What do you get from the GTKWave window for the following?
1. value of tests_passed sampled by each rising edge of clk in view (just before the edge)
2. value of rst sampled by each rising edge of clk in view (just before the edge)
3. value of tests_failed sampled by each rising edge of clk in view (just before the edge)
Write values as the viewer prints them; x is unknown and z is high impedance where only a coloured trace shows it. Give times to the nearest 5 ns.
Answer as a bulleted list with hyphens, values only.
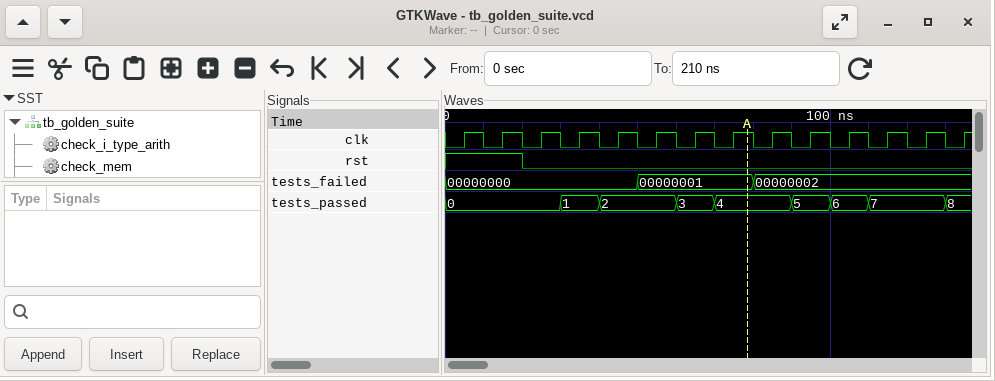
- 0, 0, 0, 1, 2, 2, 3, 4, 4, 5, 6, 7, 7, 8
- 1 1 0 0 0 0 0 0 0 0 0 0 0 0
- 00000000, 00000000, 00000000, 00000000, 00000000, 00000001, 00000001, 00000001, 00000002, 00000002, 00000002, 00000002, 00000002, 00000002
